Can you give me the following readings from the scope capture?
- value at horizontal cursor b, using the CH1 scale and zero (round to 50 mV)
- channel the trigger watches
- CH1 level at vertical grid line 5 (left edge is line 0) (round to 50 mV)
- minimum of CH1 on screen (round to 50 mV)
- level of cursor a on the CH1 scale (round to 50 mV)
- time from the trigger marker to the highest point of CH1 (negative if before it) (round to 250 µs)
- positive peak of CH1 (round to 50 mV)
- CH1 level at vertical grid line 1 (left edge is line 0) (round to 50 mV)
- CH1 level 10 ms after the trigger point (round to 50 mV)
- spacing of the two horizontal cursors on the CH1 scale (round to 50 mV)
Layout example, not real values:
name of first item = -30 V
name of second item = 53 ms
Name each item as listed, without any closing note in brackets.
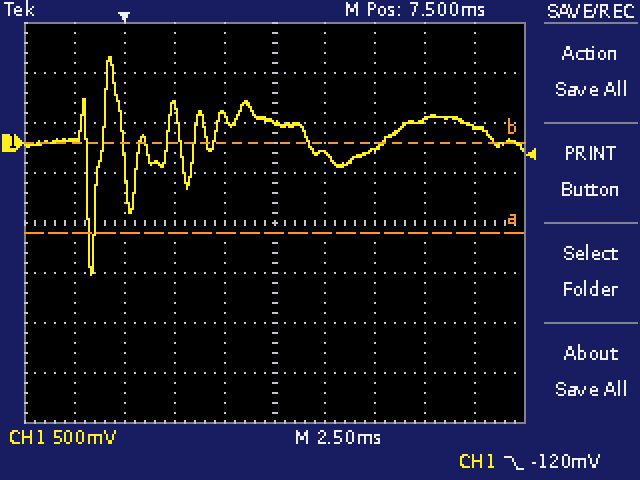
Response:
value at horizontal cursor b, using the CH1 scale and zero = 0 mV
channel the trigger watches = CH1
CH1 level at vertical grid line 5 (left edge is line 0) = 200 mV
minimum of CH1 on screen = -1.30 V
level of cursor a on the CH1 scale = -900 mV
time from the trigger marker to the highest point of CH1 (negative if before it) = -750 µs
positive peak of CH1 = 850 mV
CH1 level at vertical grid line 1 (left edge is line 0) = 50 mV
CH1 level 10 ms after the trigger point = -100 mV
spacing of the two horizontal cursors on the CH1 scale = 900 mV
